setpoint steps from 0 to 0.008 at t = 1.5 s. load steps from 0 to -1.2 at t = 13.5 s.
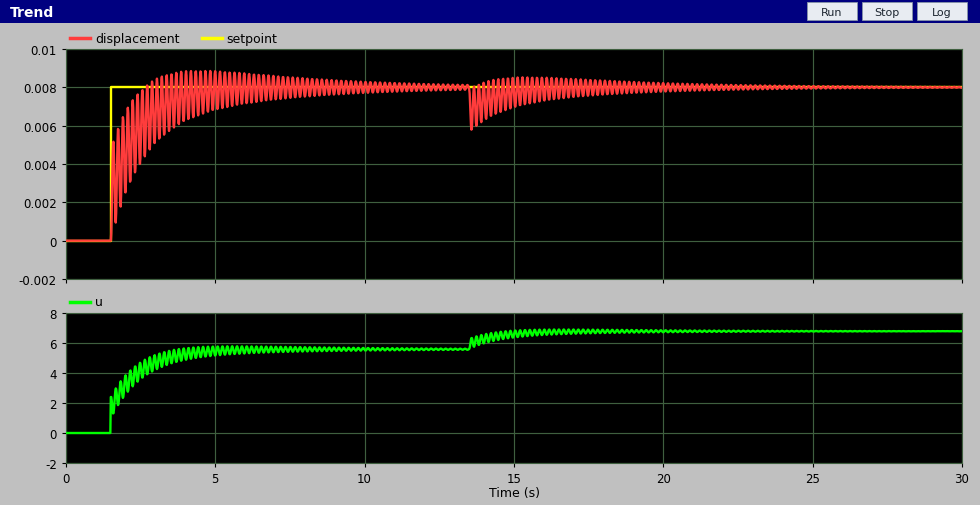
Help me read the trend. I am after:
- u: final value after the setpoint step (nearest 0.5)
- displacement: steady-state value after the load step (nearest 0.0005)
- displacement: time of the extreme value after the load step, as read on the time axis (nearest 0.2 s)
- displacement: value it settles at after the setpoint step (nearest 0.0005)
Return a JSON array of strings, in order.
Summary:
["5.5", "0.0080", "13.6 s", "0.0080"]
